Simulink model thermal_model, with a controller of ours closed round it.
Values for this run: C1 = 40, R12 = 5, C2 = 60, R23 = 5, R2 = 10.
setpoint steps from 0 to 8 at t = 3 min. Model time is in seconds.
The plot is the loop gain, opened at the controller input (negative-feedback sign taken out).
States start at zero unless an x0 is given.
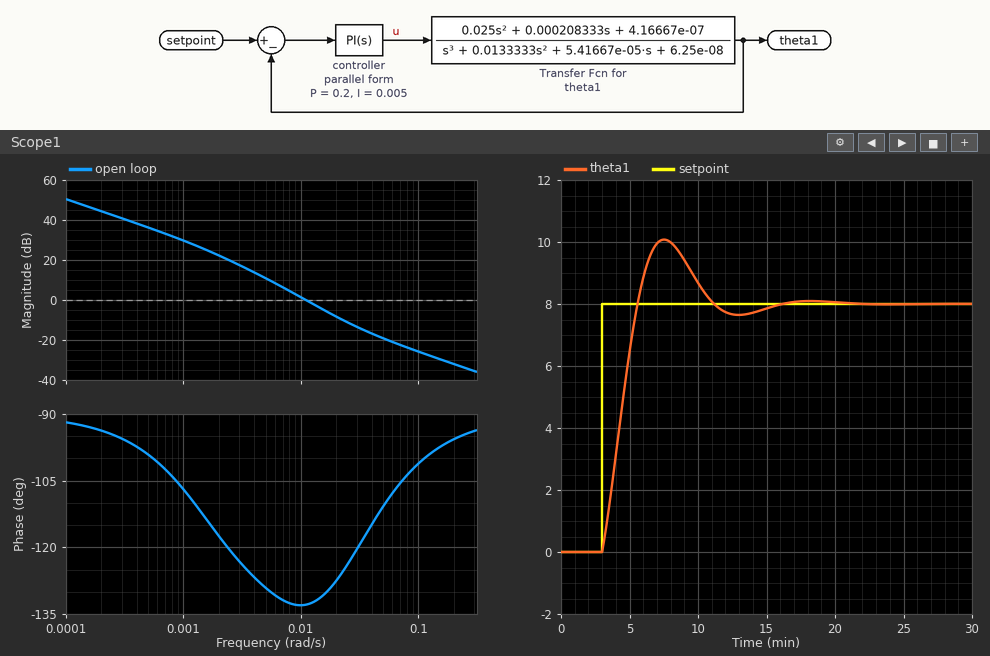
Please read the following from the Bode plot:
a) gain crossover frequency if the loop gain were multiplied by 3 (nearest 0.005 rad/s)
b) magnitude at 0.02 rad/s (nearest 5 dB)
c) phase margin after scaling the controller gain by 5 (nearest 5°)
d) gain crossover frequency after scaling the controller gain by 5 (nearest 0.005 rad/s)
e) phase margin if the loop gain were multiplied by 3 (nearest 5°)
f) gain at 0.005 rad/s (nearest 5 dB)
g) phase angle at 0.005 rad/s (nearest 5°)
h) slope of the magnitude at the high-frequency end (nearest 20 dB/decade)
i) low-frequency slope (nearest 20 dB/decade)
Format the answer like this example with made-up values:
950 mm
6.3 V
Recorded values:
0.020 rad/s
-10 dB
60°
0.030 rad/s
55°
10 dB
-130°
-20 dB/decade
-20 dB/decade
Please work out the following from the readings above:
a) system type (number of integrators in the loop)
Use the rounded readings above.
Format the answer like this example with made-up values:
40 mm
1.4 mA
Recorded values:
1
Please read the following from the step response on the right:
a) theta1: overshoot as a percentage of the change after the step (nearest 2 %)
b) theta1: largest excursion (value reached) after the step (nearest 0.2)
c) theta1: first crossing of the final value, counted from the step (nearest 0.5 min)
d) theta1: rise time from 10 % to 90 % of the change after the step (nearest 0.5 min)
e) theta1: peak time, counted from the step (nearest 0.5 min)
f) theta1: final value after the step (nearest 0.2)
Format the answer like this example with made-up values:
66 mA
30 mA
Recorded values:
26 %
10.0
2.5 min
2.0 min
4.5 min
8.0
